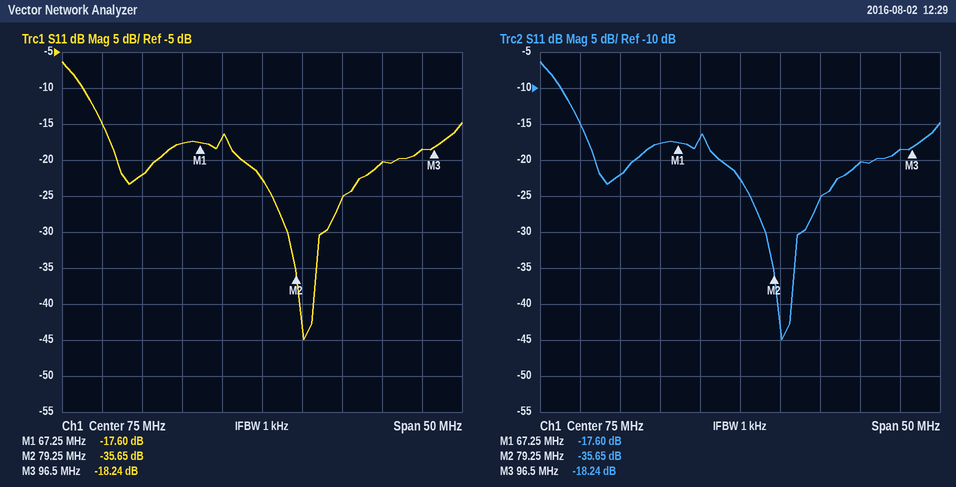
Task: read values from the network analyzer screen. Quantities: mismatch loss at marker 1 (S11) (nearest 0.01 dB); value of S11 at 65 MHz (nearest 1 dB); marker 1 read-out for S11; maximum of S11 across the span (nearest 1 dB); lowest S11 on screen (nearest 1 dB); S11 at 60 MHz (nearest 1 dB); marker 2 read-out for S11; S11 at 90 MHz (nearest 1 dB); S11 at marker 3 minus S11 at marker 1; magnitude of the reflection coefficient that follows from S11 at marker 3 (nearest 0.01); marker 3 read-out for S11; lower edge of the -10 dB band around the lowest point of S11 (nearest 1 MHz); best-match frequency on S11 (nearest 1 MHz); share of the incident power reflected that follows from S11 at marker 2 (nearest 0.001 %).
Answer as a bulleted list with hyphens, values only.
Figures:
- 0.08 dB
- -18 dB
- -17.60 dB
- -6 dB
- -45 dB
- -22 dB
- -35.65 dB
- -20 dB
- -0.64 dB
- 0.12
- -18.24 dB
- 53 MHz
- 80 MHz
- 0.027 %
